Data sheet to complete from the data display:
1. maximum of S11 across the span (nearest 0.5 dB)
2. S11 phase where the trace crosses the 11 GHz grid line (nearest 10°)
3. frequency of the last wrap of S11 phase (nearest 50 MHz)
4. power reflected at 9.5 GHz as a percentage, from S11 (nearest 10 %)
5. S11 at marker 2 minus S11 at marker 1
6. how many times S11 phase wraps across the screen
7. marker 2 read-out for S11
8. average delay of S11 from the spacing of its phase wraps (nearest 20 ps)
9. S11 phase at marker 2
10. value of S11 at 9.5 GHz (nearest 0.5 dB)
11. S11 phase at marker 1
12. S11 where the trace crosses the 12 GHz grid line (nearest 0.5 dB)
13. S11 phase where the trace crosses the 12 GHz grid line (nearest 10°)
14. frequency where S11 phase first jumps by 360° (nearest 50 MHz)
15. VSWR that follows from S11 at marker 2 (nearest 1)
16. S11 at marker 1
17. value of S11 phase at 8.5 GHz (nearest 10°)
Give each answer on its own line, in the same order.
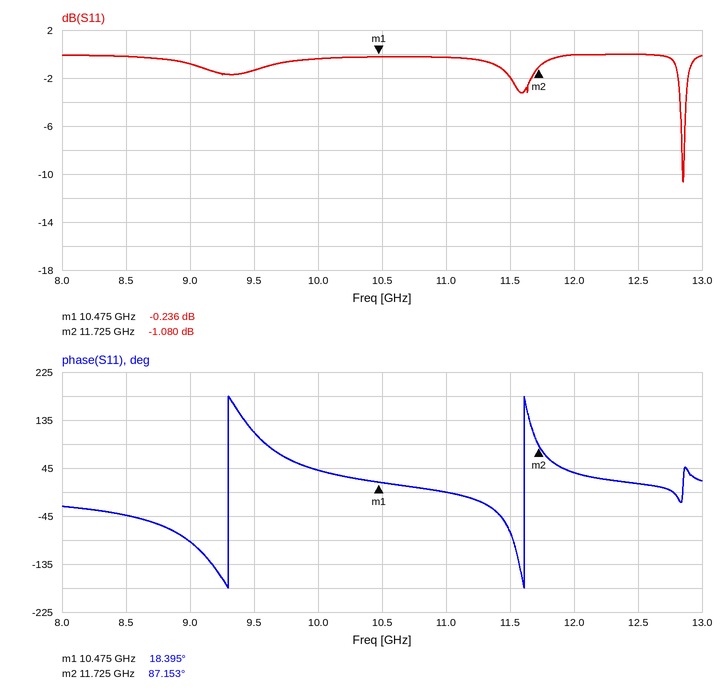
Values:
0.0 dB
0°
11.60 GHz
70 %
-0.844 dB
2
-1.080 dB
440 ps
87.153°
-1.5 dB
18.395°
0.0 dB
40°
9.30 GHz
16
-0.236 dB
-40°
